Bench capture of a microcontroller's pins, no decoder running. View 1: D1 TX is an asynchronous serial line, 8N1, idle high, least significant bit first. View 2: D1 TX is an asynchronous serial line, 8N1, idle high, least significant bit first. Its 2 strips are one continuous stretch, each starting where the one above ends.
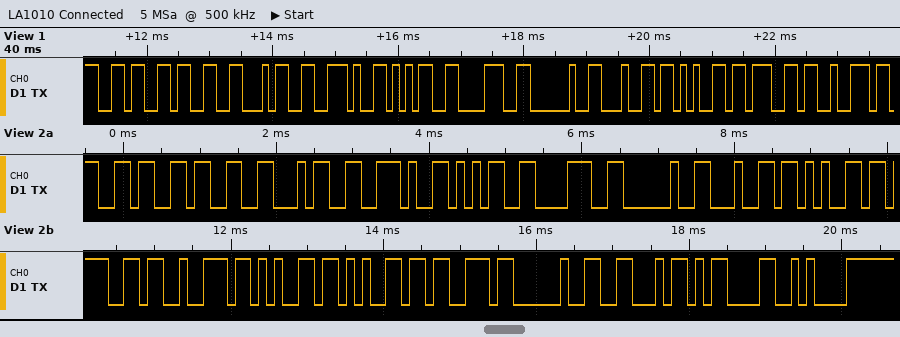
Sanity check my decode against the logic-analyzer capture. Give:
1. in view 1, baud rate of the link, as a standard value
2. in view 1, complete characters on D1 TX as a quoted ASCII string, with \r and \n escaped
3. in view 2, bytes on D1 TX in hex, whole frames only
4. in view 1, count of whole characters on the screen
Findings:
9600 baud
"634.58 degr"
36 33 34 2E 35 38 20 64 65 67 72 65 65 73 20 46 0D 0A
11
